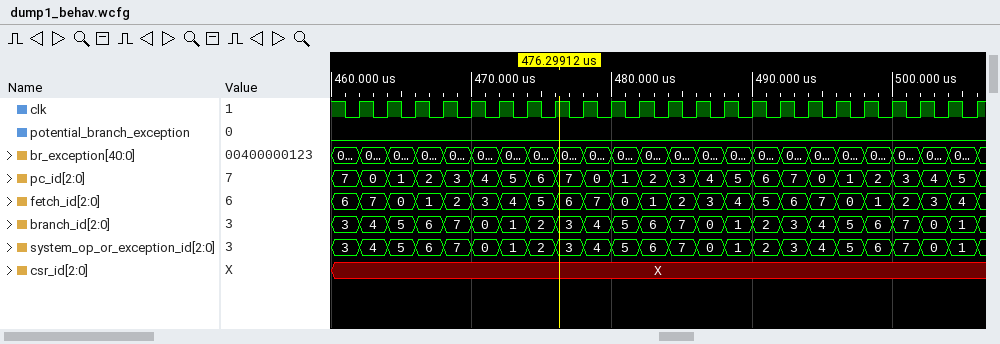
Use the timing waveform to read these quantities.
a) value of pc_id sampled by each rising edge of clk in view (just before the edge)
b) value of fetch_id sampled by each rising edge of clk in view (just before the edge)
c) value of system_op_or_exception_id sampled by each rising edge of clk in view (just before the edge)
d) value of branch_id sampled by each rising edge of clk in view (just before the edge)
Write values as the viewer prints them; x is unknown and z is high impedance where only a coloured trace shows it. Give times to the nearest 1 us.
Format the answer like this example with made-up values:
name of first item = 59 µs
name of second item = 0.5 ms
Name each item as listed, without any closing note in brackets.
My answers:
value of pc_id sampled by each rising edge of clk in view = 7, 0, 1, 2, 3, 4, 5, 6, 7, 0, 1, 2, 3, 4, 5, 6, 7, 0, 1, 2, 3, 4, 5
value of fetch_id sampled by each rising edge of clk in view = 6, 7, 0, 1, 2, 3, 4, 5, 6, 7, 0, 1, 2, 3, 4, 5, 6, 7, 0, 1, 2, 3, 4
value of system_op_or_exception_id sampled by each rising edge of clk in view = 3, 4, 5, 6, 7, 0, 1, 2, 3, 4, 5, 6, 7, 0, 1, 2, 3, 4, 5, 6, 7, 0, 1
value of branch_id sampled by each rising edge of clk in view = 3, 4, 5, 6, 7, 0, 1, 2, 3, 4, 5, 6, 7, 0, 1, 2, 3, 4, 5, 6, 7, 0, 1
